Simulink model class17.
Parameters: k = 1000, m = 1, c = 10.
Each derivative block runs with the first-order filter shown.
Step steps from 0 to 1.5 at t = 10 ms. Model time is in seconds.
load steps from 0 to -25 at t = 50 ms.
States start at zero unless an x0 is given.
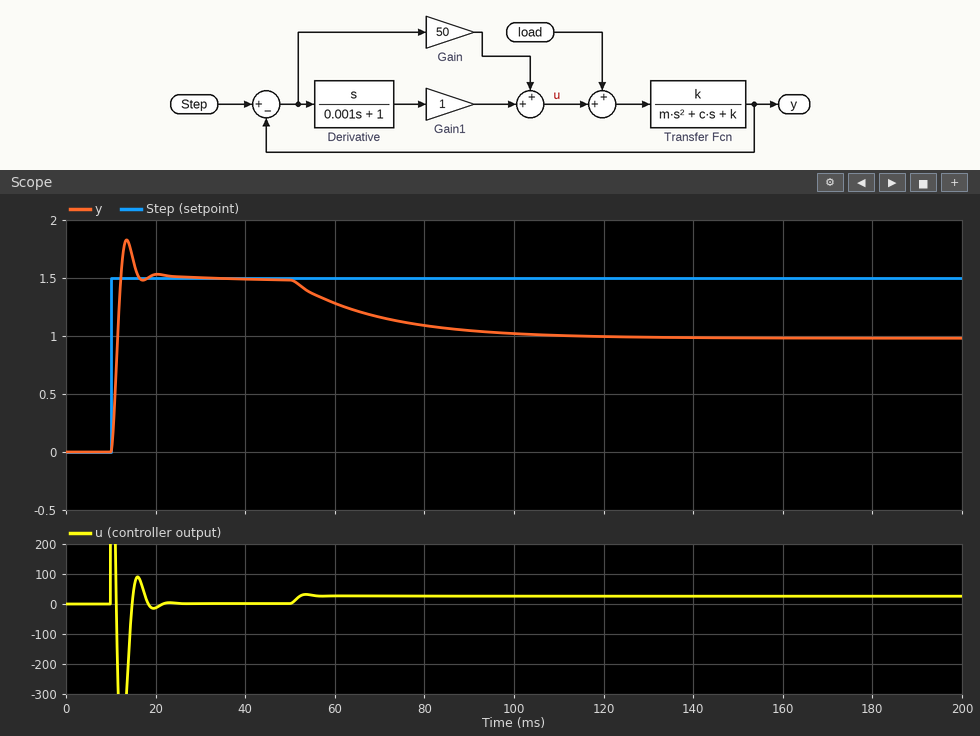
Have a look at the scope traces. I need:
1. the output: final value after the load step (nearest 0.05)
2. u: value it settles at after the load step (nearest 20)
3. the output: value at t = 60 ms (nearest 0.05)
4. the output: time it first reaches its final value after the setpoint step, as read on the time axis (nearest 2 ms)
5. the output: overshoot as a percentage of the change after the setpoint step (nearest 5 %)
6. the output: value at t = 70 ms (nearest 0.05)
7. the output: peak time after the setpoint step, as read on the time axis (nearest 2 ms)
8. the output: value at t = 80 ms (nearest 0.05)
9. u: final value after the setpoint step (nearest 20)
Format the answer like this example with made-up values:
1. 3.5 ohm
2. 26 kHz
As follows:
1. 1.00
2. 20
3. 1.30
4. 12 ms
5. 25 %
6. 1.15
7. 14 ms
8. 1.10
9. 0
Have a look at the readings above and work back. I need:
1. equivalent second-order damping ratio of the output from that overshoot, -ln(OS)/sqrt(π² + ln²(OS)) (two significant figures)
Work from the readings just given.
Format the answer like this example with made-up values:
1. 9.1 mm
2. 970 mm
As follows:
1. 0.40
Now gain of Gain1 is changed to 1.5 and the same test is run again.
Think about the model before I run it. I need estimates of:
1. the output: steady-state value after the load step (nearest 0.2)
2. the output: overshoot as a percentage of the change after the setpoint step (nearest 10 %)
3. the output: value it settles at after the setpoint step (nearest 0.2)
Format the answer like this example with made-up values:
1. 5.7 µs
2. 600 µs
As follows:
1. 1.0
2. 30 %
3. 1.4
